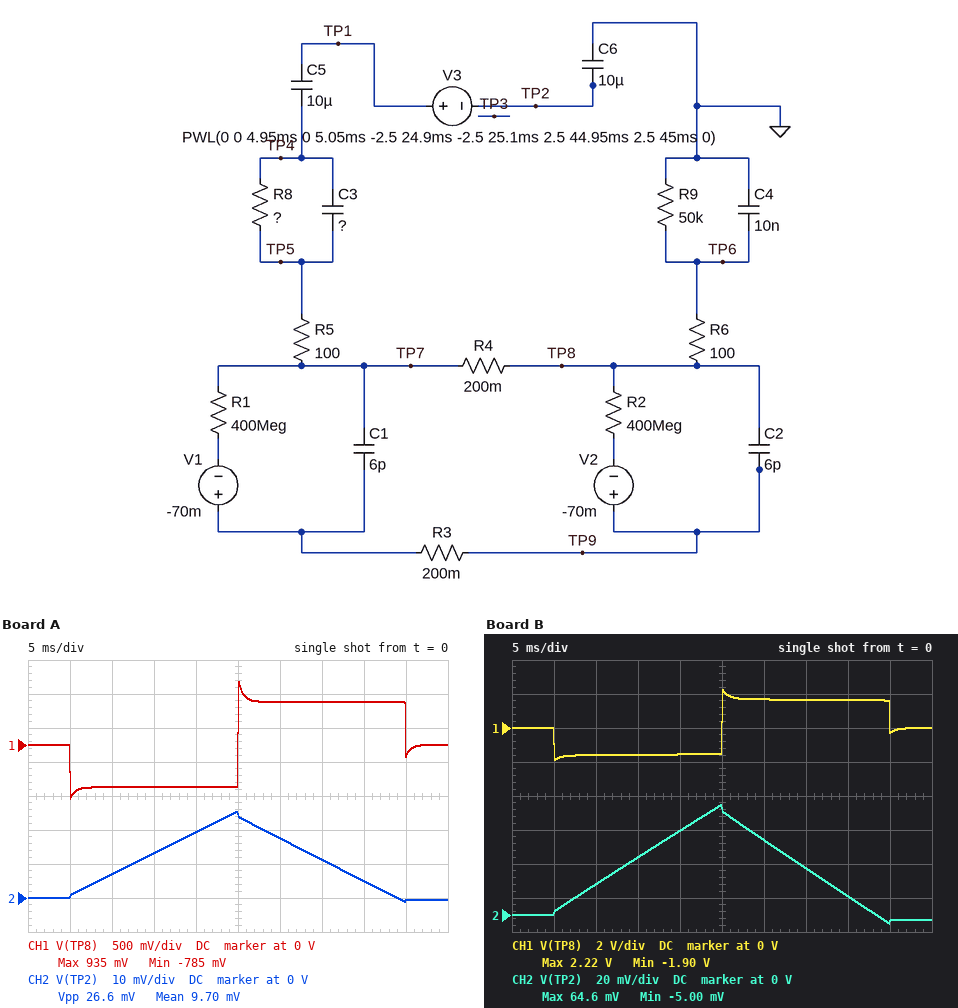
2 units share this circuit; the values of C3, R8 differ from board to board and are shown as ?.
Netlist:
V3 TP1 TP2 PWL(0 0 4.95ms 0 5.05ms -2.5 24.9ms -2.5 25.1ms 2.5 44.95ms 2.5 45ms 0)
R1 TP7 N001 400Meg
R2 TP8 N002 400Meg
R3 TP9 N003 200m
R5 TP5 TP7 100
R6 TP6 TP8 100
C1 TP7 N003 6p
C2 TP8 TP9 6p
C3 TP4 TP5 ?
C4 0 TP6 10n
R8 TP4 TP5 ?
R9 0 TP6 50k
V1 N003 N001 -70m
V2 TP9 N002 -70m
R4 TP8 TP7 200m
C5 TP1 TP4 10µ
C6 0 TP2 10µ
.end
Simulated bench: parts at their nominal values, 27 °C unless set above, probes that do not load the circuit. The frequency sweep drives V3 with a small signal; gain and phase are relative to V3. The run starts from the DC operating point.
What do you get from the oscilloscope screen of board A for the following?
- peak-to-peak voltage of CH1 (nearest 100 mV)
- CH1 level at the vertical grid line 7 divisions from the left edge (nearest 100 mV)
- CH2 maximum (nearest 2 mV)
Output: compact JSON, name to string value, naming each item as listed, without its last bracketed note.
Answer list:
{"peak-to-peak voltage of CH1": "1.7 V", "CH1 level at the vertical grid line 7 divisions from the left edge": "600 mV", "CH2 maximum": "26 mV"}
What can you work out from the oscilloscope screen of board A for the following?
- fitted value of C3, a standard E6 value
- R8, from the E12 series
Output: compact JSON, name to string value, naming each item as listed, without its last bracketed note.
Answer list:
{"fitted value of C3, a standard E6 value": "4.7 nF", "R8, from the E12 series": "150 kΩ"}
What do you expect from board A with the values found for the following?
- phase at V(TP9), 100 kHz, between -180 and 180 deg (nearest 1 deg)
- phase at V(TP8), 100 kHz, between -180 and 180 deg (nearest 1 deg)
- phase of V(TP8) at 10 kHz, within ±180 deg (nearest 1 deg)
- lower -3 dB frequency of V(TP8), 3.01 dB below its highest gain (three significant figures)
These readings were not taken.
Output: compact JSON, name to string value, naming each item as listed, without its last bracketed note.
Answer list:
{"phase at V(TP9), 100 kHz, between -180 and 180 deg": "10 deg", "phase at V(TP8), 100 kHz, between -180 and 180 deg": "10 deg", "phase of V(TP8) at 10 kHz, within ±180 deg": "2 deg", "lower -3 dB frequency of V(TP8), 3.01 dB below its highest gain": "106 kHz"}
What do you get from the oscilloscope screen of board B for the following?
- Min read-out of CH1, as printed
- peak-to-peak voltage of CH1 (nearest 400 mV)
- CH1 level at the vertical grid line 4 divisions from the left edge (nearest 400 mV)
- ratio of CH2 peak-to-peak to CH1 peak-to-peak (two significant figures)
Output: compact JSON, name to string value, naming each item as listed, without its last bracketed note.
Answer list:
{"Min read-out of CH1, as printed": "-1.90 V", "peak-to-peak voltage of CH1": "4.0 V", "CH1 level at the vertical grid line 4 divisions from the left edge": "-1.6 V", "ratio of CH2 peak-to-peak to CH1 peak-to-peak": "0.017"}
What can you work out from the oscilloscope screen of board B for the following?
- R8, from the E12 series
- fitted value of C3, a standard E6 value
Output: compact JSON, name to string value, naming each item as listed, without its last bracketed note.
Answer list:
{"R8, from the E12 series": "27 kΩ", "fitted value of C3, a standard E6 value": "33 nF"}
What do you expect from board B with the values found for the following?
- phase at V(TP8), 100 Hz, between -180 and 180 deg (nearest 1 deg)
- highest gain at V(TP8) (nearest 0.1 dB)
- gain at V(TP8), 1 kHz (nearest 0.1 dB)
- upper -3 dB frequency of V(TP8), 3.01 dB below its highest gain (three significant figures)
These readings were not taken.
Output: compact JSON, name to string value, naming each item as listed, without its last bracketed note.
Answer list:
{"phase at V(TP8), 100 Hz, between -180 and 180 deg": "4 deg", "highest gain at V(TP8)": "-2.3 dB", "gain at V(TP8), 1 kHz": "-2.4 dB", "upper -3 dB frequency of V(TP8), 3.01 dB below its highest gain": "271 kHz"}
